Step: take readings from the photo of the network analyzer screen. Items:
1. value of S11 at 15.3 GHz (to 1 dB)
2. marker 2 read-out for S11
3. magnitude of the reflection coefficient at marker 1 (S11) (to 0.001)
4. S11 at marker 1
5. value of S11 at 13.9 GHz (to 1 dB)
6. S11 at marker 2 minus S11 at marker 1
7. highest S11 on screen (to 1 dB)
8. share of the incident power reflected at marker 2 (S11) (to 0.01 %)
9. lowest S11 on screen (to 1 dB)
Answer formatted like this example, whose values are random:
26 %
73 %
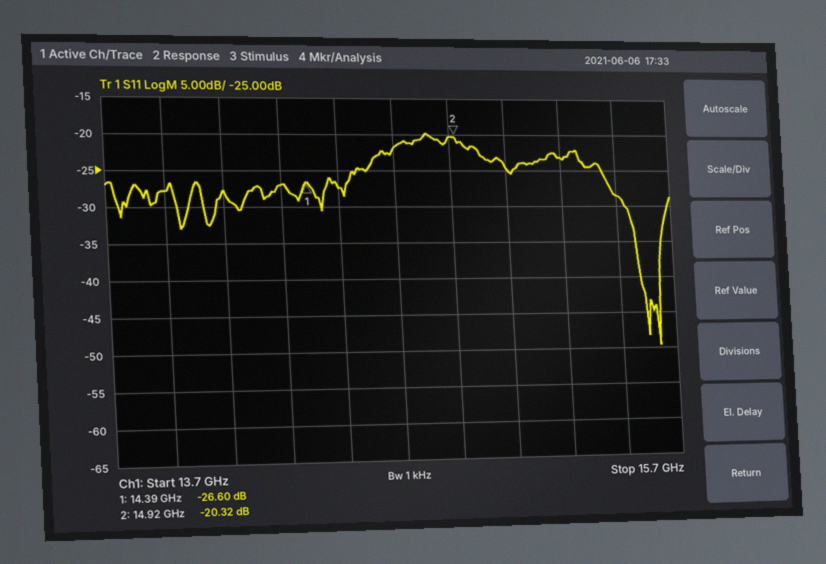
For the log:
-23 dB
-20.32 dB
0.047
-26.60 dB
-28 dB
6.28 dB
-20 dB
0.93 %
-50 dB
